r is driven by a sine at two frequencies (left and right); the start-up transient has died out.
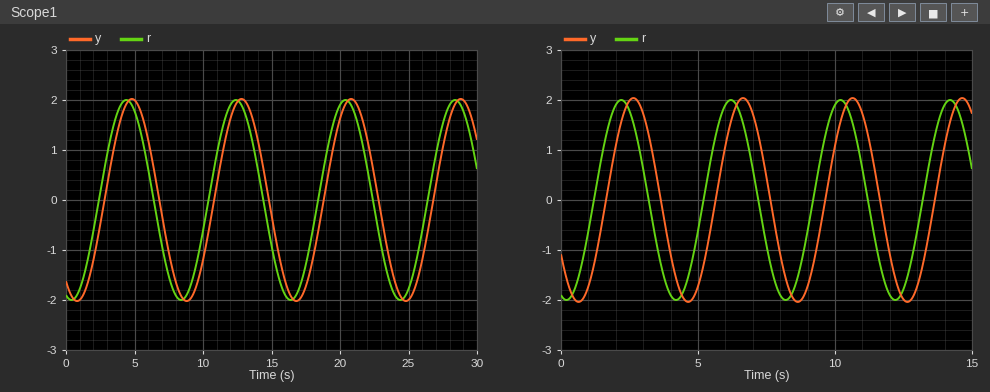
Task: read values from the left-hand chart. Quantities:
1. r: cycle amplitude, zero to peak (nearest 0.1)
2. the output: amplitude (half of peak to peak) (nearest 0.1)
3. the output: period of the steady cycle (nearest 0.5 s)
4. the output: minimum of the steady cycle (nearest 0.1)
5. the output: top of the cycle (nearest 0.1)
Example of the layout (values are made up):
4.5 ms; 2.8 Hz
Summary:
2.0; 2.0; 8.0 s; -2.0; 2.0
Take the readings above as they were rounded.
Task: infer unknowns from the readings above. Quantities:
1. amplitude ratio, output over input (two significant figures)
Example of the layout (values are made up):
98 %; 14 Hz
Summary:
1.0
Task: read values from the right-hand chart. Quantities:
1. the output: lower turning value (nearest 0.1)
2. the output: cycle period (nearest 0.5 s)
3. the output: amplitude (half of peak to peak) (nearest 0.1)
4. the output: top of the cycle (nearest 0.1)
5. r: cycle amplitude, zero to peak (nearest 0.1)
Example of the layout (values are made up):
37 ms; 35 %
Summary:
-2.0; 4.0 s; 2.0; 2.0; 2.0
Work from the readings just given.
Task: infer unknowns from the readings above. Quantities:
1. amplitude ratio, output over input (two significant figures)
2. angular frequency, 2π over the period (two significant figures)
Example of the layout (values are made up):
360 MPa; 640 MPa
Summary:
1.0; 1.6 rad/s
